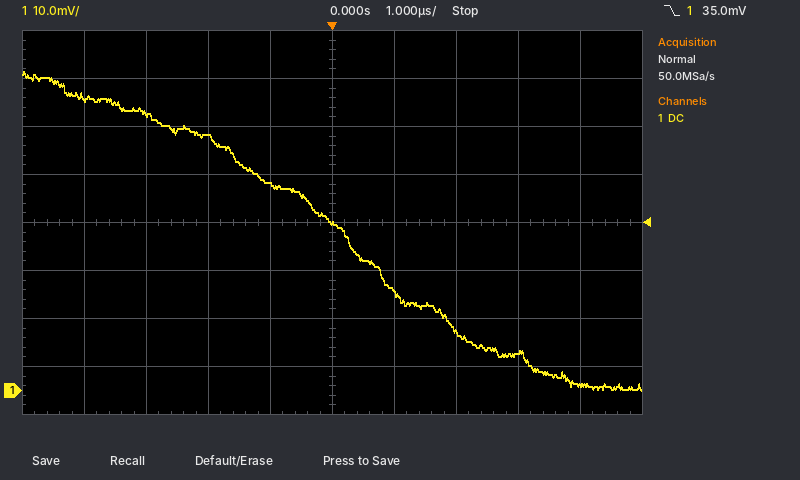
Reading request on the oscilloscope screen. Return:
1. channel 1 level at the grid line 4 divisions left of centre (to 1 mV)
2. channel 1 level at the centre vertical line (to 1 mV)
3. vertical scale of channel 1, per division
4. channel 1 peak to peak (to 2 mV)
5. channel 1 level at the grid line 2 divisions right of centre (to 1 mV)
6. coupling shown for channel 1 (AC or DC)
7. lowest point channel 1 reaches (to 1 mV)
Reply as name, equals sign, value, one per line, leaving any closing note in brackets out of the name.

channel 1 level at the grid line 4 divisions left of centre = 61 mV
channel 1 level at the centre vertical line = 35 mV
vertical scale of channel 1, per division = 10 mV
channel 1 peak to peak = 66 mV
channel 1 level at the grid line 2 divisions right of centre = 12 mV
coupling shown for channel 1 = DC
lowest point channel 1 reaches = 0 mV
